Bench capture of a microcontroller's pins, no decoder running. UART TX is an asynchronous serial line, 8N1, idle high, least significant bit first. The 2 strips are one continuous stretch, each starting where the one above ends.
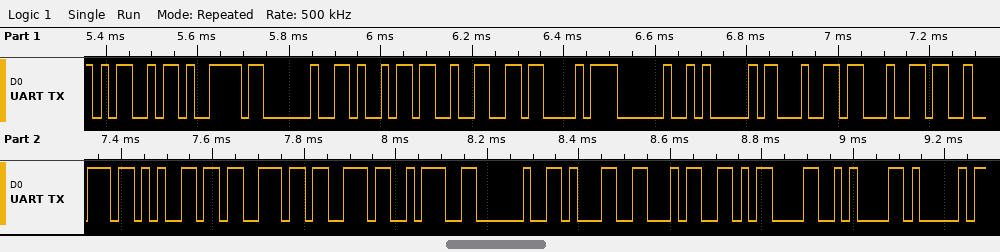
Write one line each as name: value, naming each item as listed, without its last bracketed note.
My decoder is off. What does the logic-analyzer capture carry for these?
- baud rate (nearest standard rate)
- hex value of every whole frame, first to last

baud rate: 57600 baud
hex value of every whole frame, first to last: 0x4D 0x79 0x20 0x69 0x32 0x43 0x20 0x41 0x64 0x64 0x72 0x65 0x73 0x73 0x3A 0x20 0x31 0x34 0x0D 0x0A 0x41
